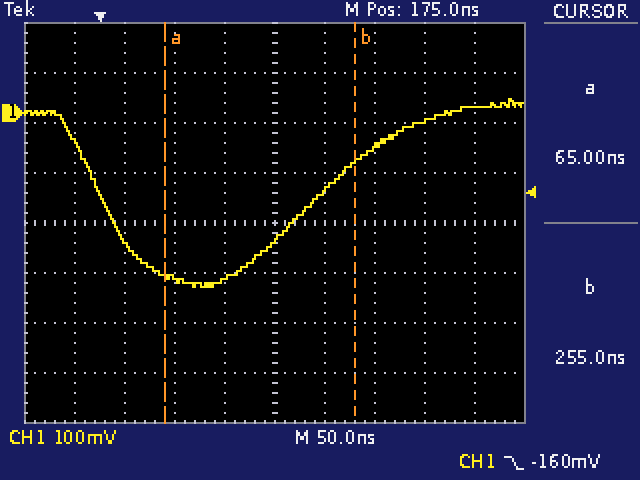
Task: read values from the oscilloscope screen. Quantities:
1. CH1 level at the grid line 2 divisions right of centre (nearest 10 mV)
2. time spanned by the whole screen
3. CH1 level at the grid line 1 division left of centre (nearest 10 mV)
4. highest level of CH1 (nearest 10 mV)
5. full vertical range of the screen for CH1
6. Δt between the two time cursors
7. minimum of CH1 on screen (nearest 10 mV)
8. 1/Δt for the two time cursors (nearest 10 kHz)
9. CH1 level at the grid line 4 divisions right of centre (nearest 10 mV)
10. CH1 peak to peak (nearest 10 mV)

-70 mV
500 ns
-330 mV
30 mV
800 mV
190 ns
-350 mV
5.26 MHz
10 mV
380 mV
